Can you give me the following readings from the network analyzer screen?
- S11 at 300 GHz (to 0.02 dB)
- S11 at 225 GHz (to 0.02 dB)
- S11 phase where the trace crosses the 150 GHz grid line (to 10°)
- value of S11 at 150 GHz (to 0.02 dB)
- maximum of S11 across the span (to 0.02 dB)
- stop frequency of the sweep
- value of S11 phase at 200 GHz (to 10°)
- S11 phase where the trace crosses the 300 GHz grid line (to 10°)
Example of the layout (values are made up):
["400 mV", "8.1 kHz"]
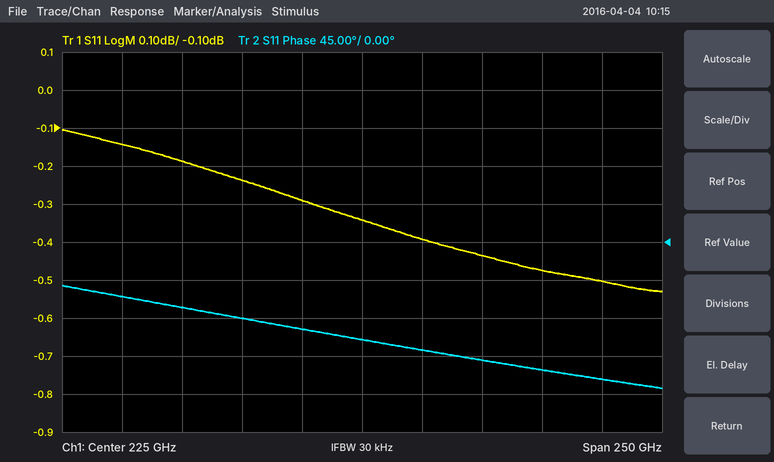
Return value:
["-0.48 dB", "-0.34 dB", "-80°", "-0.18 dB", "-0.10 dB", "350 GHz", "-100°", "-150°"]
